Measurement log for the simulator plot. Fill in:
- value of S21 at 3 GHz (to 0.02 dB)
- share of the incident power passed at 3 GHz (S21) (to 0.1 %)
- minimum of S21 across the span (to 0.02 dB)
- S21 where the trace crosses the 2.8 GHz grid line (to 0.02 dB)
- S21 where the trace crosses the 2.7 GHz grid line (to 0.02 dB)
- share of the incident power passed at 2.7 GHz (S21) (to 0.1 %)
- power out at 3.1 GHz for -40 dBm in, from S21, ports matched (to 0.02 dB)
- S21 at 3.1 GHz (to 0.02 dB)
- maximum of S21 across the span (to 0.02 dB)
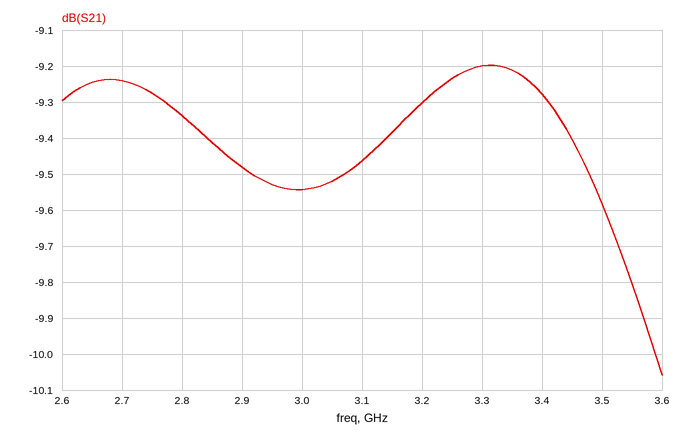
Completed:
-9.54 dB
11.1 %
-10.06 dB
-9.34 dB
-9.24 dB
11.9 %
-49.46 dBm
-9.46 dB
-9.20 dB
